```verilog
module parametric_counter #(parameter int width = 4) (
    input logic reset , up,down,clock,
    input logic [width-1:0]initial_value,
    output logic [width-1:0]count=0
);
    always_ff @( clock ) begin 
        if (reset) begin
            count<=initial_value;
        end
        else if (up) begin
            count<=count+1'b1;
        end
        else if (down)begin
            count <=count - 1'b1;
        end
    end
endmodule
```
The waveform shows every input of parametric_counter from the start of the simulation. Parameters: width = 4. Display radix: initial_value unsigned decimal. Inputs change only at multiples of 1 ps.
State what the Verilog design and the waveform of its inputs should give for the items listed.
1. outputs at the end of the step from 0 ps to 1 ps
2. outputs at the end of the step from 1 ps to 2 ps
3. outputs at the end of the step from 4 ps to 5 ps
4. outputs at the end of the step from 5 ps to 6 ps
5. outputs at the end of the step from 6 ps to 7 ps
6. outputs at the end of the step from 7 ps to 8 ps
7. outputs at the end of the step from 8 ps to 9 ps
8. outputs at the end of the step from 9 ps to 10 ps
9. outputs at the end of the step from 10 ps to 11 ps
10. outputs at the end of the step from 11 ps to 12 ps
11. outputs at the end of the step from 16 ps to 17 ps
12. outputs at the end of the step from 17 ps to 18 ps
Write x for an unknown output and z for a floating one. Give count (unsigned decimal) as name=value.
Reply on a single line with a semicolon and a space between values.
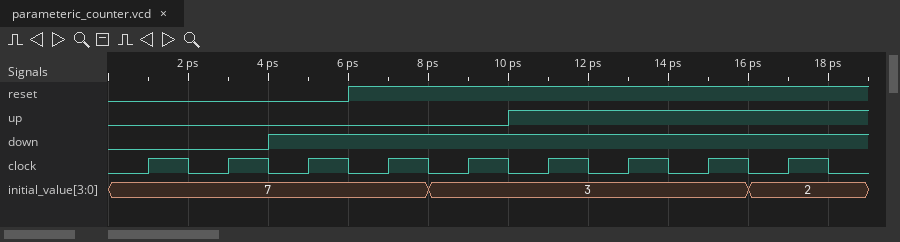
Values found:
count=0; count=0; count=15; count=14; count=7; count=7; count=3; count=3; count=3; count=3; count=2; count=2
